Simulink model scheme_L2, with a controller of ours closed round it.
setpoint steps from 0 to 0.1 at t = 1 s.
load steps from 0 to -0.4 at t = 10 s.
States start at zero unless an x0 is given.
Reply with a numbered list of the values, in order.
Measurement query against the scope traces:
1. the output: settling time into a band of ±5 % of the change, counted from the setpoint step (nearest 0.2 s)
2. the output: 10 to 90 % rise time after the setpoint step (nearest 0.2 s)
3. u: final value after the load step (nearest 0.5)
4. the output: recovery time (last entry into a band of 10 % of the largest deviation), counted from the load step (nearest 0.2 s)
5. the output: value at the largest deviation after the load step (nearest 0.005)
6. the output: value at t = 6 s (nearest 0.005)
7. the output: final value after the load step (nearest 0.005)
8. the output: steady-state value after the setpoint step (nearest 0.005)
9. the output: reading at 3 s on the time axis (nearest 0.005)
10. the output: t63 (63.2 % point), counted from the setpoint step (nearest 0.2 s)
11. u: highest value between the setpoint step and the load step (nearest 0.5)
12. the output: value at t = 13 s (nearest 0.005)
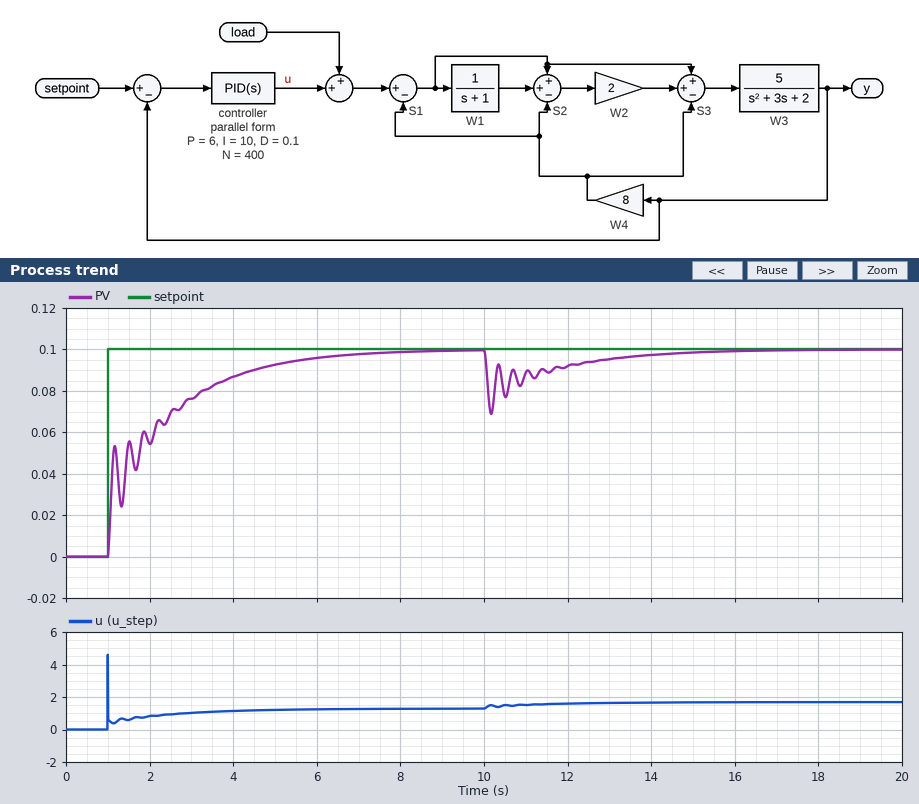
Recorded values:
1. 4.6 s
2. 3.4 s
3. 1.5
4. 3.8 s
5. 0.070
6. 0.095
7. 0.100
8. 0.100
9. 0.075
10. 1.2 s
11. 4.5
12. 0.095
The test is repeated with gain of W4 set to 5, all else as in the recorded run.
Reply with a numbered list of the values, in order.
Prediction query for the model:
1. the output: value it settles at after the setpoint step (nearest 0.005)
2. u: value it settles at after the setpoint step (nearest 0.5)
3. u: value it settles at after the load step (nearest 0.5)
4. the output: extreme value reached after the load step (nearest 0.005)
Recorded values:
1. 0.100
2. 1.0
3. 1.0
4. 0.060
